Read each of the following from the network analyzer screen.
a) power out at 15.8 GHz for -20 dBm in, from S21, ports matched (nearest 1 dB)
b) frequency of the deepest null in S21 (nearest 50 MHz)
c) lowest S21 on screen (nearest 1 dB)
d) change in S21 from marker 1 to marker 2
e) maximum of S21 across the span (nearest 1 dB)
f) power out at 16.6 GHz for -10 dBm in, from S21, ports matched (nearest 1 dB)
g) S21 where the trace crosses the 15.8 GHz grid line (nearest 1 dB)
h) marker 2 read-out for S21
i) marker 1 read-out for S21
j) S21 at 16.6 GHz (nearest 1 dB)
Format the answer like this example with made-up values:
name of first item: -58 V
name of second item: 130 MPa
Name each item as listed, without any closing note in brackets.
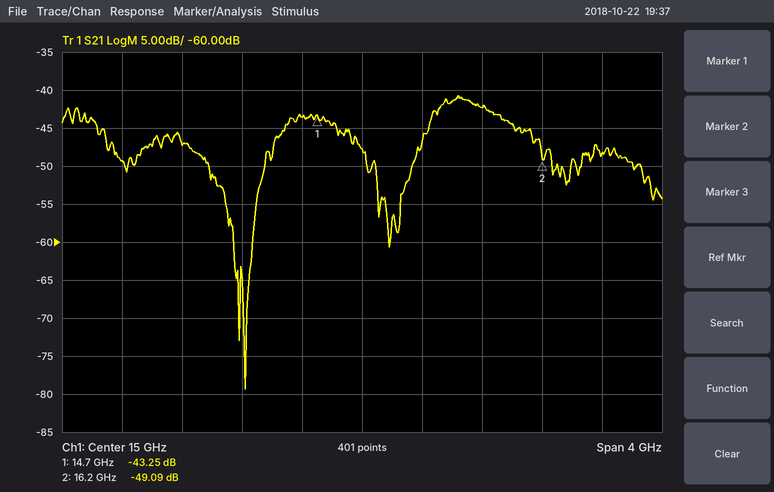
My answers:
power out at 15.8 GHz for -20 dBm in, from S21, ports matched: -62 dBm
frequency of the deepest null in S21: 14.20 GHz
lowest S21 on screen: -79 dB
change in S21 from marker 1 to marker 2: -5.84 dB
maximum of S21 across the span: -41 dB
power out at 16.6 GHz for -10 dBm in, from S21, ports matched: -58 dBm
S21 where the trace crosses the 15.8 GHz grid line: -42 dB
marker 2 read-out for S21: -49.09 dB
marker 1 read-out for S21: -43.25 dB
S21 at 16.6 GHz: -48 dB
